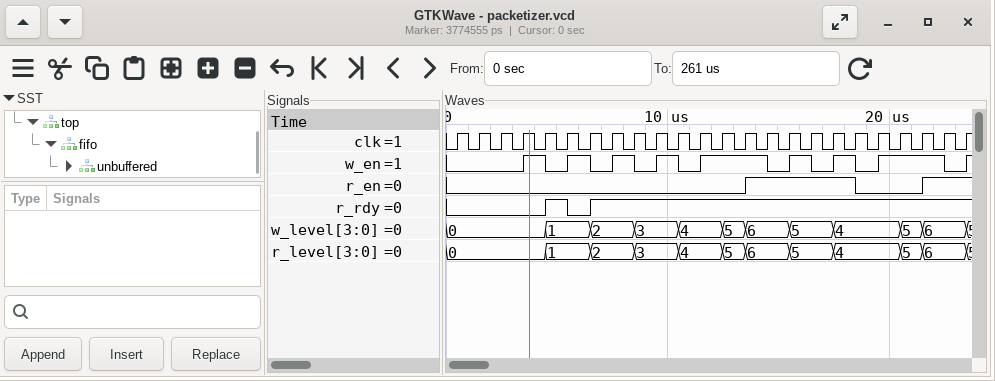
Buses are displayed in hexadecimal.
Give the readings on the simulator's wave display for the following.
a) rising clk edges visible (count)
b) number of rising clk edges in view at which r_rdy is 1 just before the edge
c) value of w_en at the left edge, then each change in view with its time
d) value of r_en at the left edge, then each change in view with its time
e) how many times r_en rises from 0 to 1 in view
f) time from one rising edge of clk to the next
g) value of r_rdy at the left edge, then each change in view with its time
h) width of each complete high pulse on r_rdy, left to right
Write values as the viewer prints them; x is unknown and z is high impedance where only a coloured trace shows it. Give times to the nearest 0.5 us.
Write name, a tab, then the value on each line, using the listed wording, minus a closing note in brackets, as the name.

rising clk edges visible	24
number of rising clk edges in view at which r_rdy is 1 just before the edge	18
value of w_en at the left edge, then each change in view with its time	0, 1 at 3.5 us, 0 at 4.5 us, 1 at 5.5 us, 0 at 6.5 us, 1 at 7.5 us, 0 at 8.5 us, 1 at 9.5 us, 0 at 10.5 us, 1 at 11.5 us, 0 at 14.5 us, 1 at 15.5 us, 0 at 16.5 us, 1 at 17.5 us, 0 at 18.5 us, 1 at 19.5 us, 0 at 22.5 us, 1 at 23.5 us
value of r_en at the left edge, then each change in view with its time	0, 1 at 13.5 us, 0 at 18.5 us, 1 at 21.5 us
how many times r_en rises from 0 to 1 in view	2
time from one rising edge of clk to the next	1 us
value of r_rdy at the left edge, then each change in view with its time	0, 1 at 4.5 us, 0 at 5.5 us, 1 at 6.5 us
width of each complete high pulse on r_rdy, left to right	1 us
